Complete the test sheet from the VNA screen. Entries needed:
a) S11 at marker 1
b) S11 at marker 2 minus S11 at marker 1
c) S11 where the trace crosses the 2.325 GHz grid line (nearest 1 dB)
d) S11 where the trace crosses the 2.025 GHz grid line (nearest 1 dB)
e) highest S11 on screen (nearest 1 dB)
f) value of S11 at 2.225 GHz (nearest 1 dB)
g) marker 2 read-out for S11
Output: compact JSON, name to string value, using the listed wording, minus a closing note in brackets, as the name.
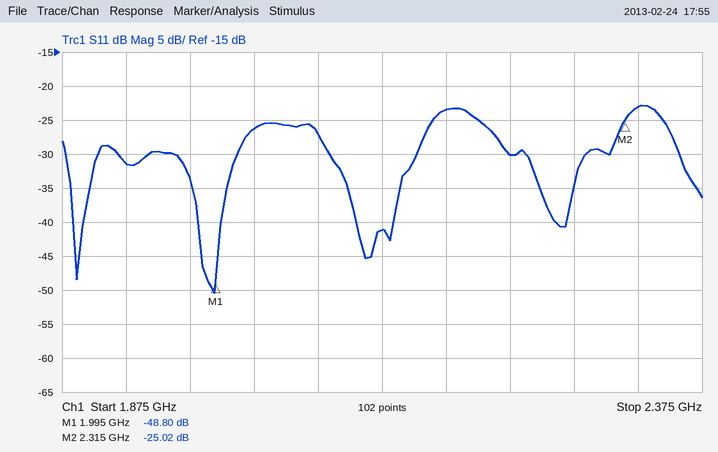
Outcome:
{"S11 at marker 1": "-48.80 dB", "S11 at marker 2 minus S11 at marker 1": "23.78 dB", "S11 where the trace crosses the 2.325 GHz grid line": "-23 dB", "S11 where the trace crosses the 2.025 GHz grid line": "-26 dB", "highest S11 on screen": "-23 dB", "value of S11 at 2.225 GHz": "-30 dB", "marker 2 read-out for S11": "-25.02 dB"}
